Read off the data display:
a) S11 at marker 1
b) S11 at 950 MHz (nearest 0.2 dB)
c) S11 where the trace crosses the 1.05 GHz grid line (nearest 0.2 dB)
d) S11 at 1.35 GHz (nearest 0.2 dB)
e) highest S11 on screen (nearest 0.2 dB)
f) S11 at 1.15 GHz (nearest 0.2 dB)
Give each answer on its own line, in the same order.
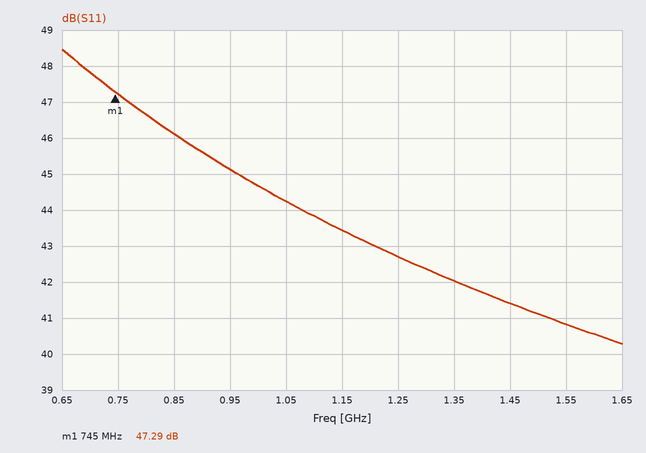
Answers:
47.29 dB
45.2 dB
44.2 dB
42.0 dB
48.4 dB
43.4 dB
